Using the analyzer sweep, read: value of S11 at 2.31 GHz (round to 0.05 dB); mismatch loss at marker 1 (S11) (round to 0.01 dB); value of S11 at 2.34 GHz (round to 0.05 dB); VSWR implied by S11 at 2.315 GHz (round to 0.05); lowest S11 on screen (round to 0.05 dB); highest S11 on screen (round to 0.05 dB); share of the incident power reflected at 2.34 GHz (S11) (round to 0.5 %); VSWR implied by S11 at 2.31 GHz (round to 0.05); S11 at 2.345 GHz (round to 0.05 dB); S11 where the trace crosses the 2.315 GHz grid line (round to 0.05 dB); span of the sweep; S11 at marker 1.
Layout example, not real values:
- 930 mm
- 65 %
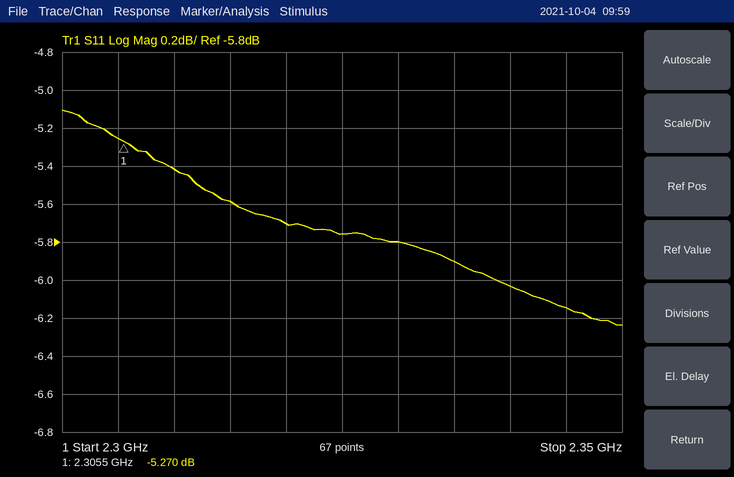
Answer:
- -5.40 dB
- 1.53 dB
- -6.05 dB
- 3.20
- -6.25 dB
- -5.10 dB
- 25.0 %
- 3.30
- -6.15 dB
- -5.60 dB
- 50 MHz
- -5.270 dB
